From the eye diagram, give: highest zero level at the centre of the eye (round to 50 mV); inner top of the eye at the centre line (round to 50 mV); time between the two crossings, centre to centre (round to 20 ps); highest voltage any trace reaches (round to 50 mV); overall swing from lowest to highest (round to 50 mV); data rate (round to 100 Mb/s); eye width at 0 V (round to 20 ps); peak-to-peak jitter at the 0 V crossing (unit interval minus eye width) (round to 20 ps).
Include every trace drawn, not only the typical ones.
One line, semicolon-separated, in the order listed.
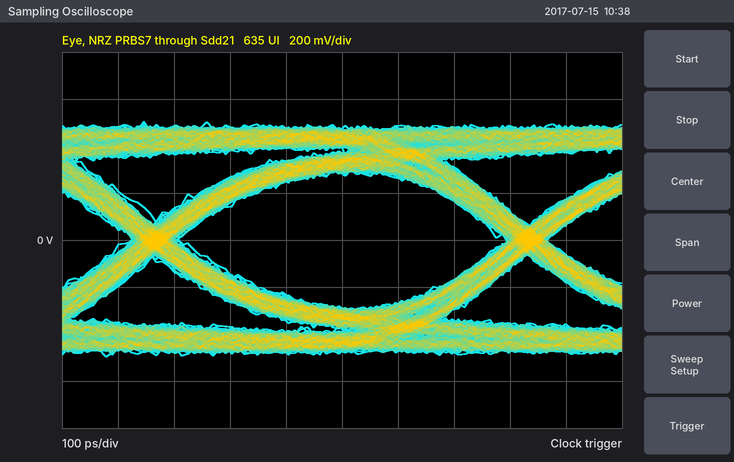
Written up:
-300 mV; 300 mV; 660 ps; 500 mV; 1.00 V; 1.5 Gb/s; 580 ps; 80 ps
